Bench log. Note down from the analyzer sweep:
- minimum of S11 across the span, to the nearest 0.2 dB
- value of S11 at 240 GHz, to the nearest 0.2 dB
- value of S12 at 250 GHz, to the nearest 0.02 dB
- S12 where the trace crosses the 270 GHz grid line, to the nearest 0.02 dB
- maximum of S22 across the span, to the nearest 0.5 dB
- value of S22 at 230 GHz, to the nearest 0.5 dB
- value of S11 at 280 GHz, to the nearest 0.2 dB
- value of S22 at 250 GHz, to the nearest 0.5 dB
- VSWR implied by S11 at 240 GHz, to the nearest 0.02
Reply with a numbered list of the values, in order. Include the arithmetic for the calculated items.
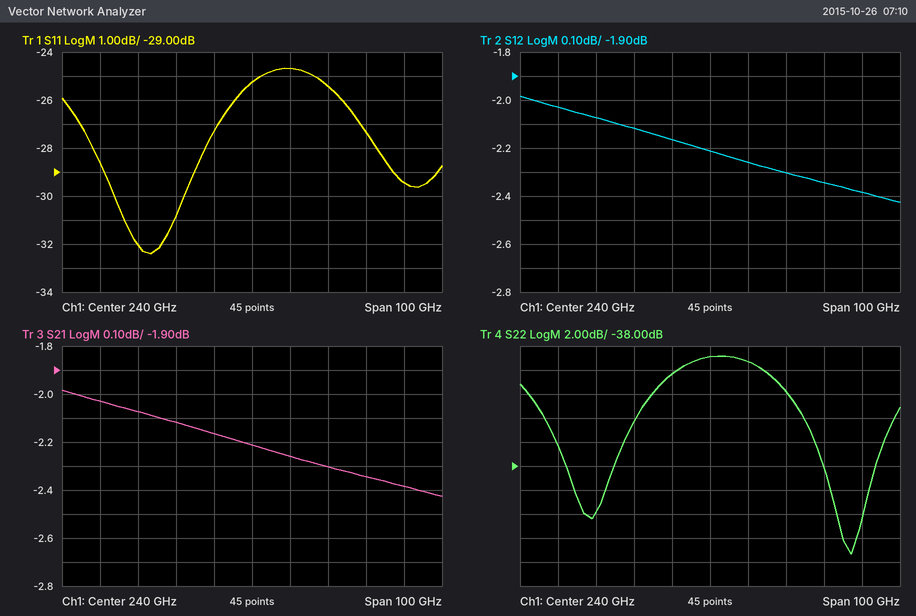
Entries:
1. -32.4 dB
2. -25.2 dB
3. -2.26 dB
4. -2.34 dB
5. -29.0 dB
6. -30.5 dB
7. -29.4 dB
8. -29.5 dB
9. |Γ| = 10^(-25.2/20) = 0.0550; VSWR = (1 + 0.0550)/(1 − 0.0550) ≈ 1.12
